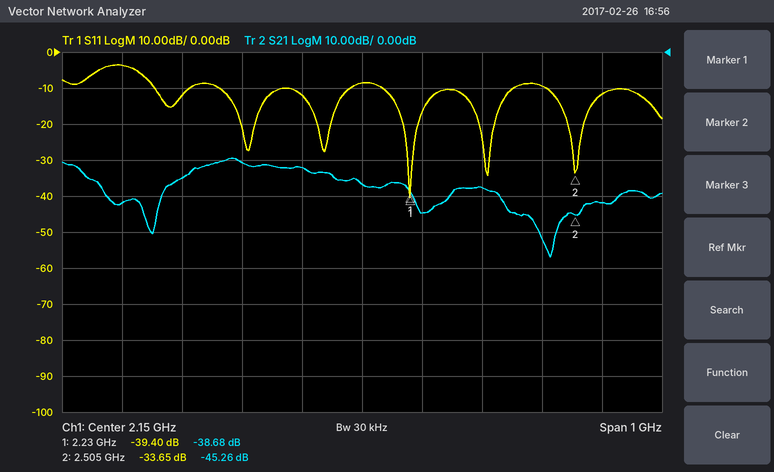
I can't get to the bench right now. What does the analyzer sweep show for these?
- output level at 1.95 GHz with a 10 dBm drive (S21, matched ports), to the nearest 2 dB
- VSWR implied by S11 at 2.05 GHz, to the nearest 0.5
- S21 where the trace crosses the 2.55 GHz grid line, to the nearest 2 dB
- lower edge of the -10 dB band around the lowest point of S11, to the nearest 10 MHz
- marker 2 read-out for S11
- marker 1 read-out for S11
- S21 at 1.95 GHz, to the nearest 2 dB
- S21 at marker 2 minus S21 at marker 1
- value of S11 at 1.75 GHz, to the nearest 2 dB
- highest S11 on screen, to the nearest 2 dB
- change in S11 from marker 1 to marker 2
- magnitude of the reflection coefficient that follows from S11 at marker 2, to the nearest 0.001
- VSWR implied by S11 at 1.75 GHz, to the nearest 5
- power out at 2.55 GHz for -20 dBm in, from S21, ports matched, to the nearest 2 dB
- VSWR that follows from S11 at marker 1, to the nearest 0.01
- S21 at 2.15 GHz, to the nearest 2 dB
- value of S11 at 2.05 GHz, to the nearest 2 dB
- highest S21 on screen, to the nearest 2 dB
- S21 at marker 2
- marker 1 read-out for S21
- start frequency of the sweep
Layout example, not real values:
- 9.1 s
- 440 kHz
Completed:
- -20 dBm
- 1.5
- -42 dB
- 2.18 GHz
- -33.65 dB
- -39.40 dB
- -30 dB
- -6.58 dB
- -4 dB
- -4 dB
- 5.75 dB
- 0.021
- 5
- -62 dBm
- 1.02
- -36 dB
- -12 dB
- -30 dB
- -45.26 dB
- -38.68 dB
- 1.65 GHz
